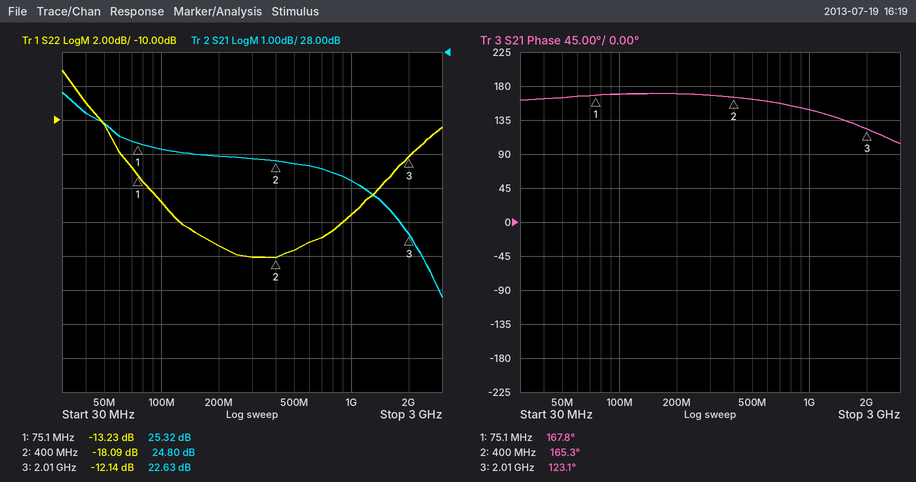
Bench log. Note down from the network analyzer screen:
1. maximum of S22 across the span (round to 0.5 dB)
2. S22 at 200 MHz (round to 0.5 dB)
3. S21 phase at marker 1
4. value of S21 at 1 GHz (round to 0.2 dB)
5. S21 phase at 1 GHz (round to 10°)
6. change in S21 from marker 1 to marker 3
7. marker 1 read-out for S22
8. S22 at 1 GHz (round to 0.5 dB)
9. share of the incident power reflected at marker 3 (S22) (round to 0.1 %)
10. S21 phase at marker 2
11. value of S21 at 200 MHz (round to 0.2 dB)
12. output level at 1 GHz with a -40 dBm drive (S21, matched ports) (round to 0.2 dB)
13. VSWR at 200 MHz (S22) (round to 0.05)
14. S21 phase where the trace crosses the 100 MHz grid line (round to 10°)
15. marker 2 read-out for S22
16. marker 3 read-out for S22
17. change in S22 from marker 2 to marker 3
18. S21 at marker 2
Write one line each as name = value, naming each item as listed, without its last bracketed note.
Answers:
maximum of S22 across the span = -7.0 dB
S22 at 200 MHz = -17.5 dB
S21 phase at marker 1 = 167.8°
value of S21 at 1 GHz = 24.2 dB
S21 phase at 1 GHz = 150°
change in S21 from marker 1 to marker 3 = -2.69 dB
marker 1 read-out for S22 = -13.23 dB
S22 at 1 GHz = -15.5 dB
share of the incident power reflected at marker 3 (S22) = 6.1 %
S21 phase at marker 2 = 165.3°
value of S21 at 200 MHz = 25.0 dB
output level at 1 GHz with a -40 dBm drive (S21, matched ports) = -15.8 dBm
VSWR at 200 MHz (S22) = 1.30
S21 phase where the trace crosses the 100 MHz grid line = 170°
marker 2 read-out for S22 = -18.09 dB
marker 3 read-out for S22 = -12.14 dB
change in S22 from marker 2 to marker 3 = 5.95 dB
S21 at marker 2 = 24.80 dB
